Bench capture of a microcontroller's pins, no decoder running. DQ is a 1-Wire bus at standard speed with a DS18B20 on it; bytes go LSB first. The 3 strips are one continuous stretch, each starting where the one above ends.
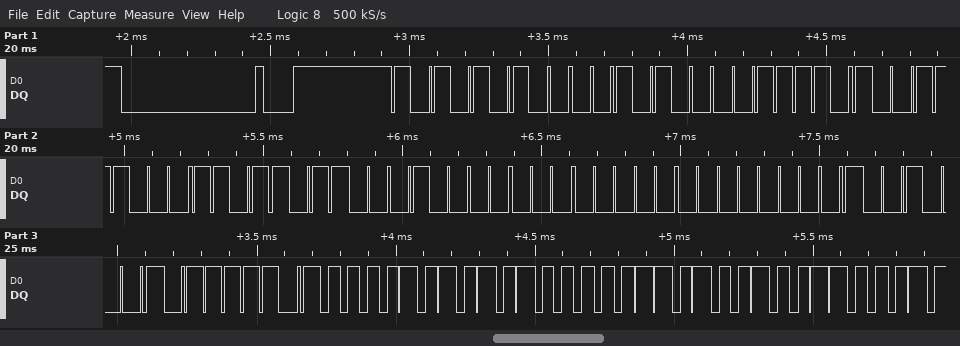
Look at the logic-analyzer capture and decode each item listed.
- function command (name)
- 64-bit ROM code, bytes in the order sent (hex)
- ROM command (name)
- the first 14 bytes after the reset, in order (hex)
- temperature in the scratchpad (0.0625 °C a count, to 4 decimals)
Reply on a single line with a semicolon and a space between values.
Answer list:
Read Scratchpad; 28 BC 1C DB 08 00 00 89; Match ROM; 55 28 BC 1C DB 08 00 00 89 BE 50 05 4B 46; 85.0000 °C
